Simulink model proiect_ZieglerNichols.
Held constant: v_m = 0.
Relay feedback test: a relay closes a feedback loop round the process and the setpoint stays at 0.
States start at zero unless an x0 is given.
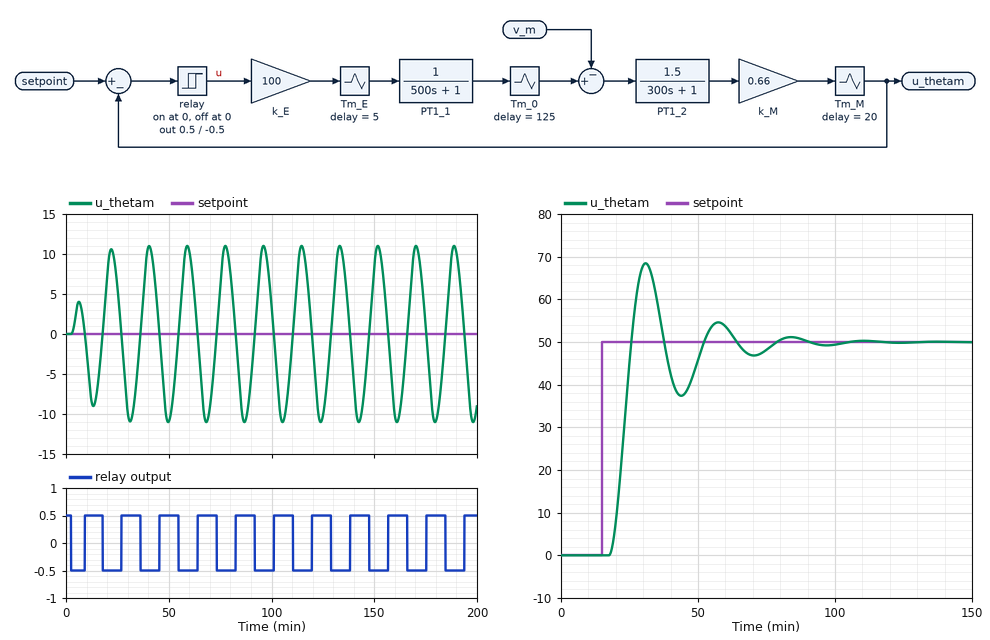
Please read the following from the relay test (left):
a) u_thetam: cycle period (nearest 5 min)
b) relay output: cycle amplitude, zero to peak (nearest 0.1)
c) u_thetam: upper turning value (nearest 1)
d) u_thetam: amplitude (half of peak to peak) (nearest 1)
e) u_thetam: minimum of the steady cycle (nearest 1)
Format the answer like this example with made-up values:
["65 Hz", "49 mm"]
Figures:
["20 min", "0.5", "11", "11", "-11"]
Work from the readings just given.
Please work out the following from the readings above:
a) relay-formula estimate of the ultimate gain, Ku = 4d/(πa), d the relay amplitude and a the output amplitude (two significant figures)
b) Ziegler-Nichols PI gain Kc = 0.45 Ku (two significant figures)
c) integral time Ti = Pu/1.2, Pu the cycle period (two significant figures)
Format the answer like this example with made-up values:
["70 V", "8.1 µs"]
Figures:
["0.058", "0.026", "17 min"]
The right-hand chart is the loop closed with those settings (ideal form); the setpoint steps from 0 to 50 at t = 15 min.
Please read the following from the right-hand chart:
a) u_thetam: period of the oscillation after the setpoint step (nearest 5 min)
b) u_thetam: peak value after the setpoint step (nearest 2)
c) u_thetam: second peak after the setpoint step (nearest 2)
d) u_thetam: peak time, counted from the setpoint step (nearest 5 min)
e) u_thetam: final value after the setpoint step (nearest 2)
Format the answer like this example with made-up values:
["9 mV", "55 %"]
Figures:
["25 min", "68", "54", "15 min", "50"]
